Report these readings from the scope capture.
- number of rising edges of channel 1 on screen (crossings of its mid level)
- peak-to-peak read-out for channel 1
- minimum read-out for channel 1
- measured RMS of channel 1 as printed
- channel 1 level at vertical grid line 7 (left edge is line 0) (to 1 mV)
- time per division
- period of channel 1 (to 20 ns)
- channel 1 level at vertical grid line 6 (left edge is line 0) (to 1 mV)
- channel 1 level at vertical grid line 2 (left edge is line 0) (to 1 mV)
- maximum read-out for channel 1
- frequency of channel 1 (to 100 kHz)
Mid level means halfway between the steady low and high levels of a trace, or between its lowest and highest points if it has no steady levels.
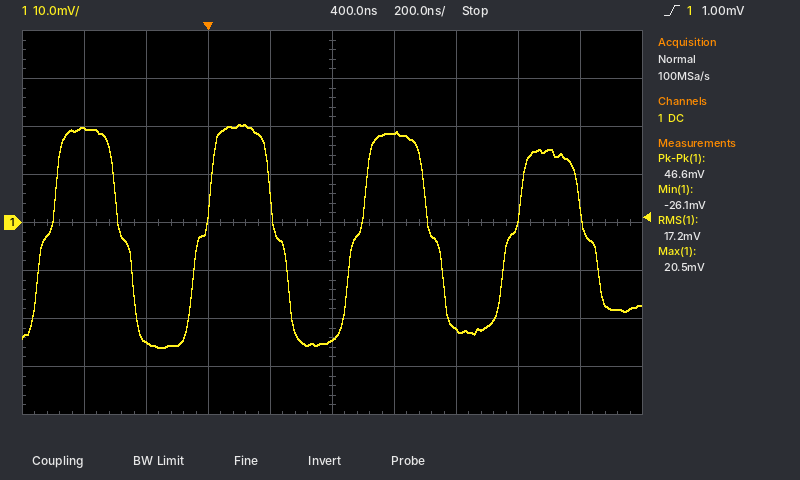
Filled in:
4
46.6 mV
-26.1 mV
17.2 mV
-22 mV
200 ns
500 ns
19 mV
-25 mV
20.5 mV
2.0 MHz
